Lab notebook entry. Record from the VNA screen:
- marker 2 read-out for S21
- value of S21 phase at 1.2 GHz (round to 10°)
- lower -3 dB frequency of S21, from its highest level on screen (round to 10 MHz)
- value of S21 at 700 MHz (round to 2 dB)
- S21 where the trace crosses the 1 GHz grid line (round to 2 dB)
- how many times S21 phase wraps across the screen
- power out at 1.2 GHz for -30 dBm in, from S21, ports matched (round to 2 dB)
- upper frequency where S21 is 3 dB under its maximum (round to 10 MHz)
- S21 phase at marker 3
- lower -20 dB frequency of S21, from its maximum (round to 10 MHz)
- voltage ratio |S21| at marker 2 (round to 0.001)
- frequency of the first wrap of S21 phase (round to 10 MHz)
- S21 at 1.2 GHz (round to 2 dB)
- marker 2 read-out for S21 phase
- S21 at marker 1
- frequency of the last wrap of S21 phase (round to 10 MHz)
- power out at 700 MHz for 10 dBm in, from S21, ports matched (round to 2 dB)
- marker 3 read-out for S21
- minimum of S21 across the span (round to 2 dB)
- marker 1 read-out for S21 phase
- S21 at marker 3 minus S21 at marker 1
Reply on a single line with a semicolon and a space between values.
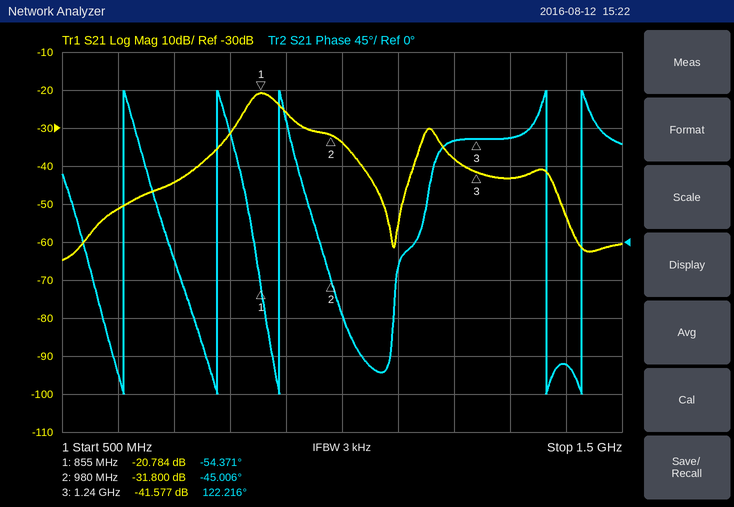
-31.800 dB; 120°; 830 MHz; -44 dB; -34 dB; 5; -68 dBm; 890 MHz; 122.216°; 740 MHz; 0.026; 610 MHz; -38 dB; -45.006°; -20.784 dB; 1.43 GHz; -34 dBm; -41.577 dB; -64 dB; -54.371°; -20.793 dB
